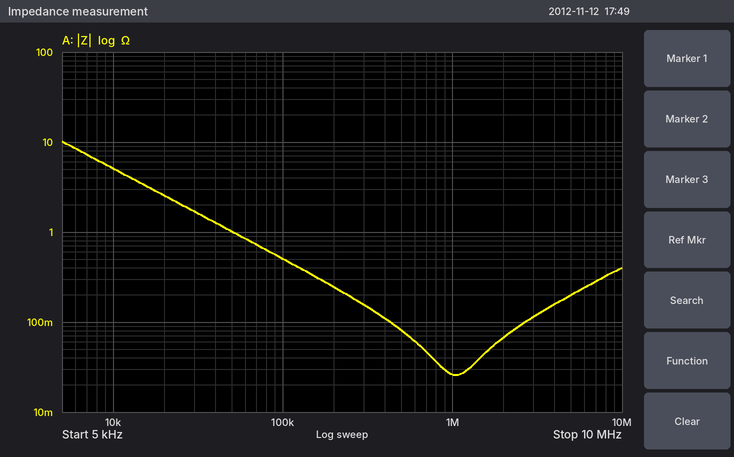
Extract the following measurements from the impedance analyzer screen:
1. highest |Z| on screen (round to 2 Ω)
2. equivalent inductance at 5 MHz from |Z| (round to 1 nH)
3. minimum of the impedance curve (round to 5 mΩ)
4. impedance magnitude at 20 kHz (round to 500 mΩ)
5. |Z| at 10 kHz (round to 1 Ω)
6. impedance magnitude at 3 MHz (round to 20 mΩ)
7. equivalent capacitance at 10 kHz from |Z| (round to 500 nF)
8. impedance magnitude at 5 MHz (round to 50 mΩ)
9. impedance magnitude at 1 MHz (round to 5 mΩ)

10 Ω
6 nH
25 mΩ
2.5 Ω
5 Ω
120 mΩ
3.0 µF
200 mΩ
25 mΩ
